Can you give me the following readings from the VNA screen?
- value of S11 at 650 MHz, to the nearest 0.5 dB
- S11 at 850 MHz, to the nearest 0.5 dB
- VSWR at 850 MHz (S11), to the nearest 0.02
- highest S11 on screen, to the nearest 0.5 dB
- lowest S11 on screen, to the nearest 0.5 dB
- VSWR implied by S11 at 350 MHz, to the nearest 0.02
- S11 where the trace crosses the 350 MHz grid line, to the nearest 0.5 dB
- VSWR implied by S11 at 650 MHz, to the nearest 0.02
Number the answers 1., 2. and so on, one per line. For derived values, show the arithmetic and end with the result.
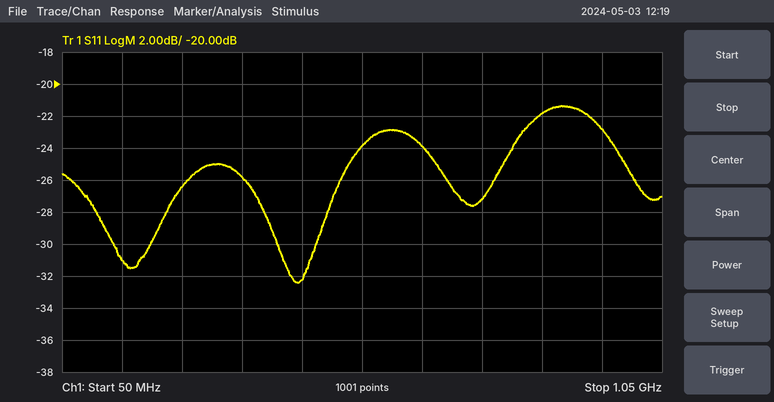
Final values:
1. -24.0 dB
2. -22.0 dB
3. |Γ| = 10^(-22/20) = 0.0794; VSWR = (1 + 0.0794)/(1 − 0.0794) ≈ 1.17, so 1.18 to the nearest 0.02
4. -21.5 dB
5. -32.5 dB
6. |Γ| = 10^(-26/20) = 0.0501; VSWR = (1 + 0.0501)/(1 − 0.0501) ≈ 1.11, so 1.10 to the nearest 0.02
7. -26.0 dB
8. |Γ| = 10^(-24/20) = 0.0631; VSWR = (1 + 0.0631)/(1 − 0.0631) ≈ 1.13, so 1.14 to the nearest 0.02
